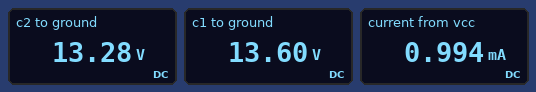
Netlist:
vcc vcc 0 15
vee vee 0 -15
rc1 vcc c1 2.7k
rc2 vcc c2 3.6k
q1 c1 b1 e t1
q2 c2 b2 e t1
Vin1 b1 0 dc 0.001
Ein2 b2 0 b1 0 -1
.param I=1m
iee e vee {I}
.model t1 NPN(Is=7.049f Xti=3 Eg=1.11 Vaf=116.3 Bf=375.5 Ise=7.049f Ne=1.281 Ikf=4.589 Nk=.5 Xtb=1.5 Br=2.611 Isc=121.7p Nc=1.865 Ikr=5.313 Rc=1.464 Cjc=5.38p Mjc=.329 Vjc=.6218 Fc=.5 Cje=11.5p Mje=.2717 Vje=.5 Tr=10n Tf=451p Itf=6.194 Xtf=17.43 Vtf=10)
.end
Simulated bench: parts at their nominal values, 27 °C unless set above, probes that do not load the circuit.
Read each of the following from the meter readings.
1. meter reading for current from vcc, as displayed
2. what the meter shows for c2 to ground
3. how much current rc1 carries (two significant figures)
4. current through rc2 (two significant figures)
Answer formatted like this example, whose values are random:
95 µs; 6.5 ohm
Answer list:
0.994 mA; 13.28 V; 520 µA; 480 µA
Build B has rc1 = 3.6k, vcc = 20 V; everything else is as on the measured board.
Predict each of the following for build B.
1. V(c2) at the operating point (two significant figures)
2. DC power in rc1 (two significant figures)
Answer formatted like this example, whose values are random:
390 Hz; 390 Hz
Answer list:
18 V; 960 µW
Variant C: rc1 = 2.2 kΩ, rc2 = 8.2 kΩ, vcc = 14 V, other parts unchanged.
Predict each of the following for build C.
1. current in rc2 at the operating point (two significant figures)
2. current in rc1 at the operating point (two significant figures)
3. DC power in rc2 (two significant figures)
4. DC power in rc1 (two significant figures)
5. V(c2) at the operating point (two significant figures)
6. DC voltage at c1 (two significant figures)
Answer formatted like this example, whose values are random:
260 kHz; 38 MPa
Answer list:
470 µA; 520 µA; 1.8 mW; 600 µW; 10 V; 13 V
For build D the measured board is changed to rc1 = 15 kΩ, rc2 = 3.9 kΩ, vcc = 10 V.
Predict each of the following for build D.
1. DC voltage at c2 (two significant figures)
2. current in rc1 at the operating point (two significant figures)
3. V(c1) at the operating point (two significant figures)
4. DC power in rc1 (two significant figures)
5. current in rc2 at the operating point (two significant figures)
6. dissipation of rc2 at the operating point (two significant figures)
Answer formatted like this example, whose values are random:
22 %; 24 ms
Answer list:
8.1 V; 500 µA; 2.4 V; 3.8 mW; 490 µA; 930 µW
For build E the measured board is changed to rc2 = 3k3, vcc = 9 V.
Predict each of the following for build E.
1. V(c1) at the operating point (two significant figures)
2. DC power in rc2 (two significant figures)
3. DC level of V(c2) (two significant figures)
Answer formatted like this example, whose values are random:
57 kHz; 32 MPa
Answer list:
7.6 V; 750 µW; 7.4 V
